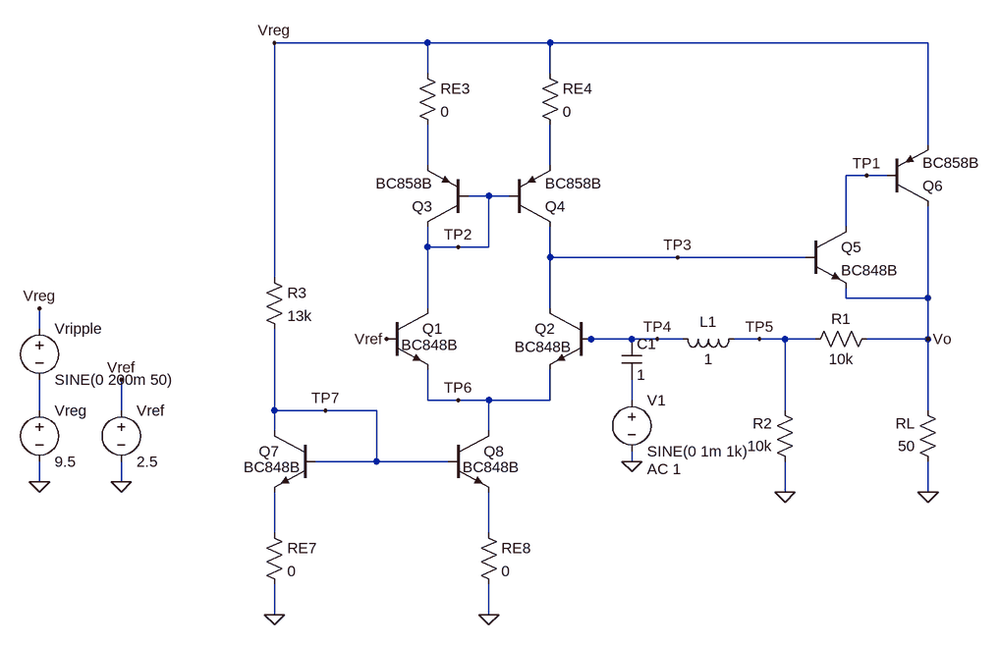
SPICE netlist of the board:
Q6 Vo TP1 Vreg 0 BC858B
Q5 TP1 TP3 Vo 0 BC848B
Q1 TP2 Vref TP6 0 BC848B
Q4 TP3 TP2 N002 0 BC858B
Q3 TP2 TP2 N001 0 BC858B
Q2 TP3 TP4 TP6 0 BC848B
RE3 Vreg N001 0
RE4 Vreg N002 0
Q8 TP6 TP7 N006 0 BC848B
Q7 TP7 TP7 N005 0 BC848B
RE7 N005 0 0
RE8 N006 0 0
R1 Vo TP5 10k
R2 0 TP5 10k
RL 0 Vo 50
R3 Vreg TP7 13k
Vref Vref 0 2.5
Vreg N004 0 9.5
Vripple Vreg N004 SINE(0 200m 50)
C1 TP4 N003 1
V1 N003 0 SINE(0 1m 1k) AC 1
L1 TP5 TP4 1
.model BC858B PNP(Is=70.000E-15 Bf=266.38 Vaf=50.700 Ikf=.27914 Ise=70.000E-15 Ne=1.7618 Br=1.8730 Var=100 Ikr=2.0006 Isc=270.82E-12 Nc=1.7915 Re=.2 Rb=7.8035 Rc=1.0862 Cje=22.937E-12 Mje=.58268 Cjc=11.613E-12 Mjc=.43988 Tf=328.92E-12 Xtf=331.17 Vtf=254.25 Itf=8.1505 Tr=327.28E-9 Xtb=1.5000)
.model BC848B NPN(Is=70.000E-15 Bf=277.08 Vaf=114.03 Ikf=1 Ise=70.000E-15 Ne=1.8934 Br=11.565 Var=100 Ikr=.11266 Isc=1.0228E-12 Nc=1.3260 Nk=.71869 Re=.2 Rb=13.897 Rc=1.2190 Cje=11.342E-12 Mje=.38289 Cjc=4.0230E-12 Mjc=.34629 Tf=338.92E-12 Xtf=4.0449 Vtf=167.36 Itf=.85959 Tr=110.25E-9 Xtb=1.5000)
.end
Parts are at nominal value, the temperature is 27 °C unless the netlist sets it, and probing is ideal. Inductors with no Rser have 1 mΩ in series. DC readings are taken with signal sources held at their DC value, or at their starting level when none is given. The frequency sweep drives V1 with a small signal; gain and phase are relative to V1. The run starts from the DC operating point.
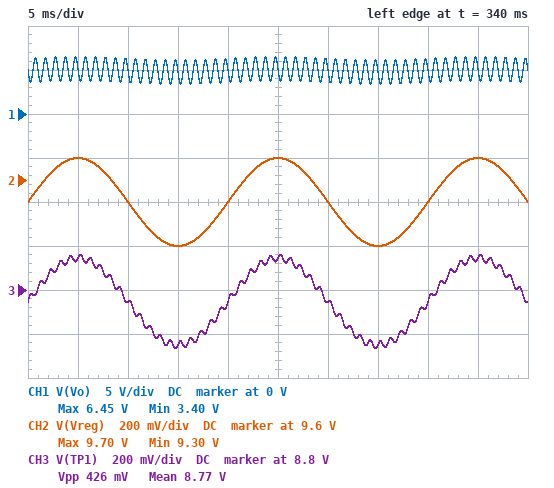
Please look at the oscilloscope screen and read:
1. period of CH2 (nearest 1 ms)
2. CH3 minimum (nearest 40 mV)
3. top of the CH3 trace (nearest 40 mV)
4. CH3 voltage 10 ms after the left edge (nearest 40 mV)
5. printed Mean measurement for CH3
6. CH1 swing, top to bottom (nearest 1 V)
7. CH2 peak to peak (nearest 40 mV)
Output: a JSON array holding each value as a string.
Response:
["20 ms", "8.52 V", "8.96 V", "8.76 V", "8.77 V", "3 V", "400 mV"]
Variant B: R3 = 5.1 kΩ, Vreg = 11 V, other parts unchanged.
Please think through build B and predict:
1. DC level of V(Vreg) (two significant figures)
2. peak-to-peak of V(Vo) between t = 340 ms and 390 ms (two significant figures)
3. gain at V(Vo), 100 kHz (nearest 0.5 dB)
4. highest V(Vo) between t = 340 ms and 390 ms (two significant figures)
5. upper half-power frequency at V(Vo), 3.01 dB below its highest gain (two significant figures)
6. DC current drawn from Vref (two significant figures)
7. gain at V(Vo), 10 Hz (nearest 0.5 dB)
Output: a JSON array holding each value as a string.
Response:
["11 V", "3.2 V", "62.5 dB", "6.6 V", "260 kHz", "3.3 µA", "63.0 dB"]
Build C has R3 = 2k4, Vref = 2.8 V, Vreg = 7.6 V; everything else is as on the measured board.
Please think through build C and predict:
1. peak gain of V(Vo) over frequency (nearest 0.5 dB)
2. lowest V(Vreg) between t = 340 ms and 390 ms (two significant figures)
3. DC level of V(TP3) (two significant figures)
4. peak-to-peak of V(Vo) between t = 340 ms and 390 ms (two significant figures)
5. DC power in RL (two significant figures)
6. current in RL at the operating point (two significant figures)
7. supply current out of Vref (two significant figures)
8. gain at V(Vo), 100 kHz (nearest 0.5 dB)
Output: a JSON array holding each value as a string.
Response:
["62.5 dB", "7.4 V", "6.2 V", "2.8 V", "640 mW", "110 mA", "5.1 µA", "62.0 dB"]
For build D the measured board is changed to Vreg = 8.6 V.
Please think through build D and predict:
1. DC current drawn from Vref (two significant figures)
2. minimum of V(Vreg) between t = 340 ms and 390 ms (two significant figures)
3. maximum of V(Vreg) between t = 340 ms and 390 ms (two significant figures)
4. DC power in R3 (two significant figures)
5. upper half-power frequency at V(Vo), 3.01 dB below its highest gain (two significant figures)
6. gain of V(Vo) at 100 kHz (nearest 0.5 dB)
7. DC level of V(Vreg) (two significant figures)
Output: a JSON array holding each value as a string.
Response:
["1.1 µA", "8.4 V", "8.8 V", "4.9 mW", "78 kHz", "58.0 dB", "8.6 V"]
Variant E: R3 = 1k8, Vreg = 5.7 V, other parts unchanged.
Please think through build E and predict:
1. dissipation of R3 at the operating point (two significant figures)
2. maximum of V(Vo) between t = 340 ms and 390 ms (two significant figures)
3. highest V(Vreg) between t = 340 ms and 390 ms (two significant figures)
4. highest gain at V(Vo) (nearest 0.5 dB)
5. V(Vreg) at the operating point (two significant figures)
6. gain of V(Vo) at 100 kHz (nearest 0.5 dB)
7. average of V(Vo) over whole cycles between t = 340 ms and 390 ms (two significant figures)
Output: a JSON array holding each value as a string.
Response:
["14 mW", "5.1 V", "5.9 V", "-28.5 dB", "5.7 V", "-31.5 dB", "4.9 V"]
